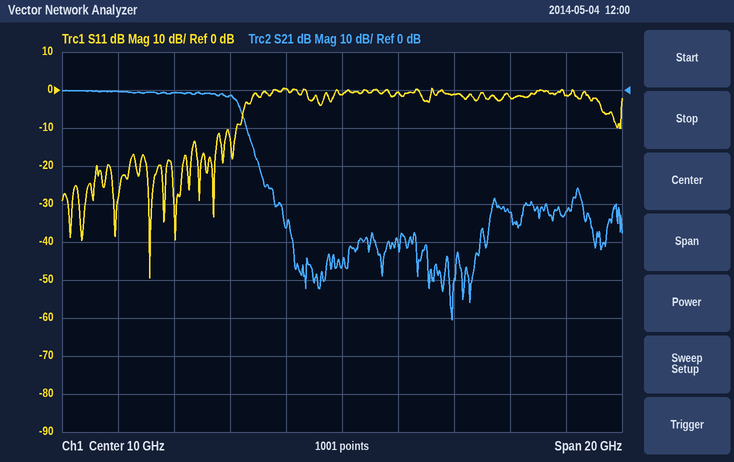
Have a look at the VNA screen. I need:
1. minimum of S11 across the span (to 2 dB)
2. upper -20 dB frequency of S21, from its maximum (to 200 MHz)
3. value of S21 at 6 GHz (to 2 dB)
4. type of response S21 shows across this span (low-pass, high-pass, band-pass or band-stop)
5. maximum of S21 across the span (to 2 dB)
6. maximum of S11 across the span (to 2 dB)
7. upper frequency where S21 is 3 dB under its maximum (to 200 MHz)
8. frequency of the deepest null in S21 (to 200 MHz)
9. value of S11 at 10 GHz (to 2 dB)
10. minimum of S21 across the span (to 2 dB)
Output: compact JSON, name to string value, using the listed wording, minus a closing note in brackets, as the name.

{"minimum of S11 across the span": "-50 dB", "upper -20 dB frequency of S21, from its maximum": "7.0 GHz", "value of S21 at 6 GHz": "-2 dB", "type of response S21 shows across this span": "low-pass", "maximum of S21 across the span": "0 dB", "maximum of S11 across the span": "0 dB", "upper frequency where S21 is 3 dB under its maximum": "6.2 GHz", "frequency of the deepest null in S21": "14.0 GHz", "value of S11 at 10 GHz": "-2 dB", "minimum of S21 across the span": "-60 dB"}
